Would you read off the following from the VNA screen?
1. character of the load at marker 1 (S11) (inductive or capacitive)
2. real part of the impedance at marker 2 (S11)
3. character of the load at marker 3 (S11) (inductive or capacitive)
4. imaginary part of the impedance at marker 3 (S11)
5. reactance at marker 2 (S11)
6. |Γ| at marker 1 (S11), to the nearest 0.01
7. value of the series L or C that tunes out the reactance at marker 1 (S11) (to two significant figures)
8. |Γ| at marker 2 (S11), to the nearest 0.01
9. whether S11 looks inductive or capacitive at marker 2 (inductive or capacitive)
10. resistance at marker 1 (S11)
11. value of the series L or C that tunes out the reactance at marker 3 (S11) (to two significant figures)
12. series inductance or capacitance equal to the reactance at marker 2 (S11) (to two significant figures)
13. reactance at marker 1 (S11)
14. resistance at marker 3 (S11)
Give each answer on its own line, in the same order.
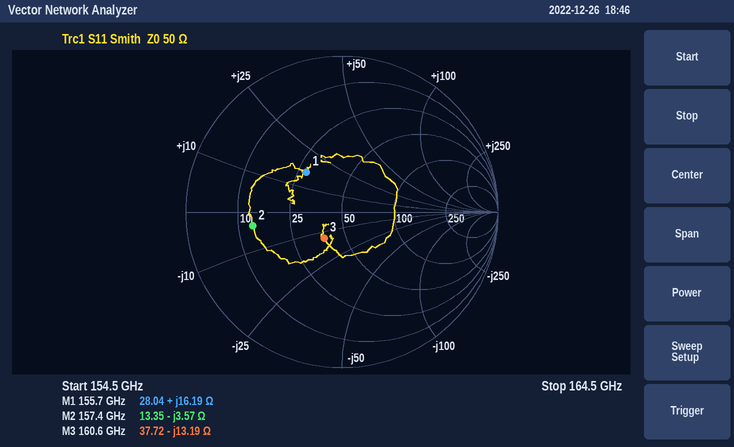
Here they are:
inductive
13.35 Ω
capacitive
-13.19 Ω
-3.57 Ω
0.34
63 fF
0.58
capacitive
28.04 Ω
13 pH
280 fF
+16.19 Ω
37.72 Ω
